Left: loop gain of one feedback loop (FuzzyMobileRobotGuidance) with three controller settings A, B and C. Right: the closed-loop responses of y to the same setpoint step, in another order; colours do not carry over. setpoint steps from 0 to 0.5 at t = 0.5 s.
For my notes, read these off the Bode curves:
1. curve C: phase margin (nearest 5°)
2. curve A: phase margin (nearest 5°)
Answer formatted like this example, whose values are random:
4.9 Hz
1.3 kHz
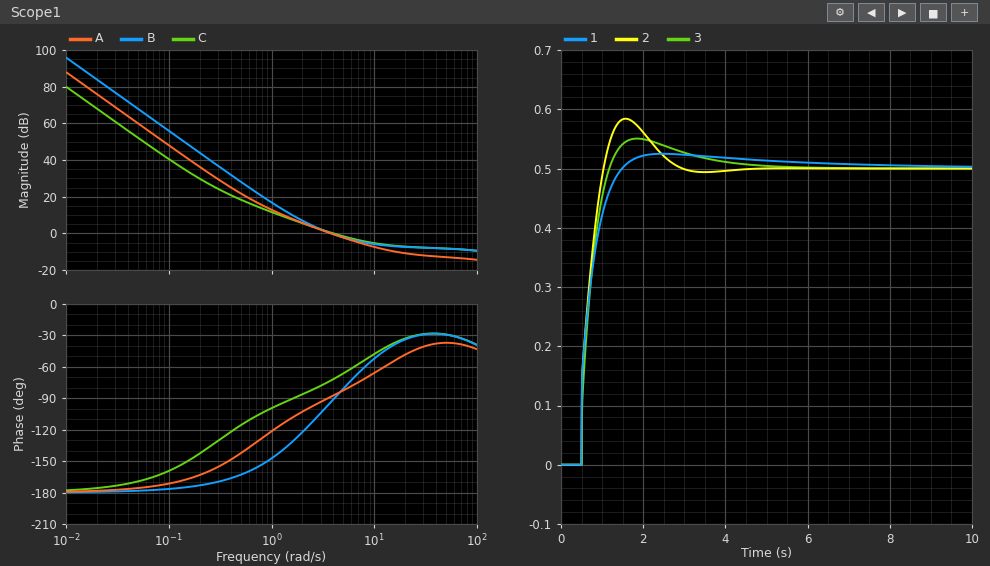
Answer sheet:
110°
90°
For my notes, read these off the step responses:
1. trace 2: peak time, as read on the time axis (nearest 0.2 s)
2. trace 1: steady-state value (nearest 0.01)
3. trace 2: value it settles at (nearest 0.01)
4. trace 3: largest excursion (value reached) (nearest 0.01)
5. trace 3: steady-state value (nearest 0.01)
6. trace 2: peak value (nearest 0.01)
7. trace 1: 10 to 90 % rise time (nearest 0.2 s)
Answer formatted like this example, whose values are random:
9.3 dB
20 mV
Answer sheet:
1.6 s
0.50
0.50
0.55
0.50
0.58
0.6 s
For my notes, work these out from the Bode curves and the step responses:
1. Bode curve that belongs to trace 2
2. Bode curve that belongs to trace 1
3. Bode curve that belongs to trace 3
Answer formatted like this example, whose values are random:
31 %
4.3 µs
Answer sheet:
B
C
A
